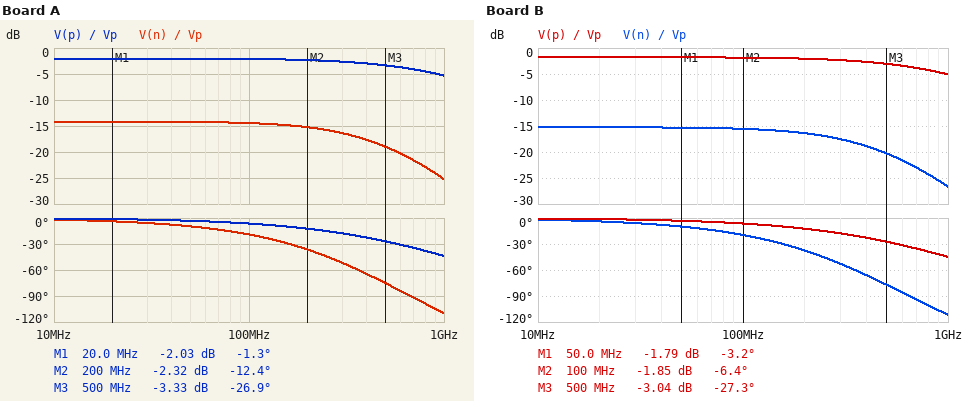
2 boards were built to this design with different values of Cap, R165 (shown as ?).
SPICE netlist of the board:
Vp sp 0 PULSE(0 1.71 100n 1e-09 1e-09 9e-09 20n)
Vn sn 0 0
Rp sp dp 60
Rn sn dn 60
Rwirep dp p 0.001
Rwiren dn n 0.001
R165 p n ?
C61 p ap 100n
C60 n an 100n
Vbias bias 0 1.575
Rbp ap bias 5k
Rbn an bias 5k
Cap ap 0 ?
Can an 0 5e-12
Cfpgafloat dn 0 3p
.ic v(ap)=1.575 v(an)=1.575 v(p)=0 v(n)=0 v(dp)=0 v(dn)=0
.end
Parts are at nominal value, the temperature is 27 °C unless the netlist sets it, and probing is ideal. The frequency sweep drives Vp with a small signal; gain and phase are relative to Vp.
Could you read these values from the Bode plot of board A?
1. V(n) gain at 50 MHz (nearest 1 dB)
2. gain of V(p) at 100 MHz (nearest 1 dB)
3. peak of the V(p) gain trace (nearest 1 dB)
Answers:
-14 dB
-2 dB
-2 dB
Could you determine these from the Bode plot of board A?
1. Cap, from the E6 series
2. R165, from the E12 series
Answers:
3.3 pF
180 Ω
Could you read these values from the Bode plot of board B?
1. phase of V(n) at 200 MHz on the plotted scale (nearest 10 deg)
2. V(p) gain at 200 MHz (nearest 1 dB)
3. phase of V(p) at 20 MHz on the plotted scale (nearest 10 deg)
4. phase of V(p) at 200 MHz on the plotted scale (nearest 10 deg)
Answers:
-40 deg
-2 dB
0 deg
-10 deg
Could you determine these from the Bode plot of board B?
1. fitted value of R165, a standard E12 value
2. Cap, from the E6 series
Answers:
220 Ω
3.3 pF
